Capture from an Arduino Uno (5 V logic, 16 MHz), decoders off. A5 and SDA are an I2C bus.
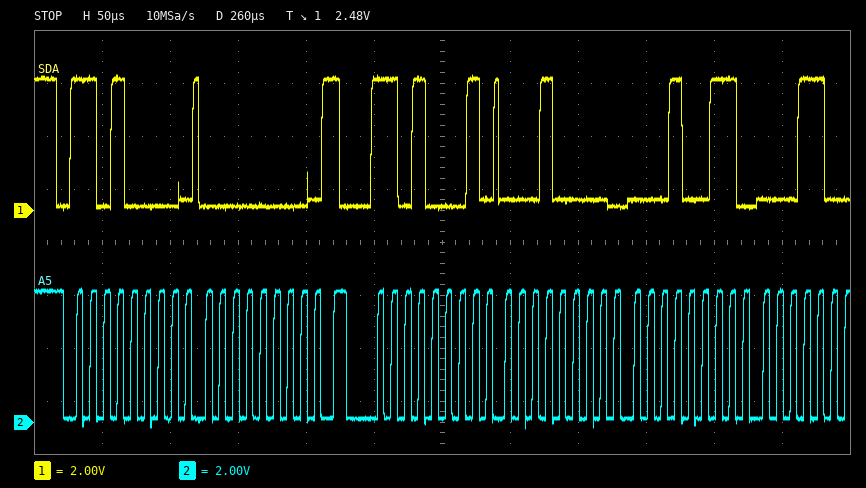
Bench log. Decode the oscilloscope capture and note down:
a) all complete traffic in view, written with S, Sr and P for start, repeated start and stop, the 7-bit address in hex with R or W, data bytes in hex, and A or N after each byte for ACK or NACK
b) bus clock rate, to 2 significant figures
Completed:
S 68W A 00 A Sr 68R A 10 A 13 A
100 kHz
